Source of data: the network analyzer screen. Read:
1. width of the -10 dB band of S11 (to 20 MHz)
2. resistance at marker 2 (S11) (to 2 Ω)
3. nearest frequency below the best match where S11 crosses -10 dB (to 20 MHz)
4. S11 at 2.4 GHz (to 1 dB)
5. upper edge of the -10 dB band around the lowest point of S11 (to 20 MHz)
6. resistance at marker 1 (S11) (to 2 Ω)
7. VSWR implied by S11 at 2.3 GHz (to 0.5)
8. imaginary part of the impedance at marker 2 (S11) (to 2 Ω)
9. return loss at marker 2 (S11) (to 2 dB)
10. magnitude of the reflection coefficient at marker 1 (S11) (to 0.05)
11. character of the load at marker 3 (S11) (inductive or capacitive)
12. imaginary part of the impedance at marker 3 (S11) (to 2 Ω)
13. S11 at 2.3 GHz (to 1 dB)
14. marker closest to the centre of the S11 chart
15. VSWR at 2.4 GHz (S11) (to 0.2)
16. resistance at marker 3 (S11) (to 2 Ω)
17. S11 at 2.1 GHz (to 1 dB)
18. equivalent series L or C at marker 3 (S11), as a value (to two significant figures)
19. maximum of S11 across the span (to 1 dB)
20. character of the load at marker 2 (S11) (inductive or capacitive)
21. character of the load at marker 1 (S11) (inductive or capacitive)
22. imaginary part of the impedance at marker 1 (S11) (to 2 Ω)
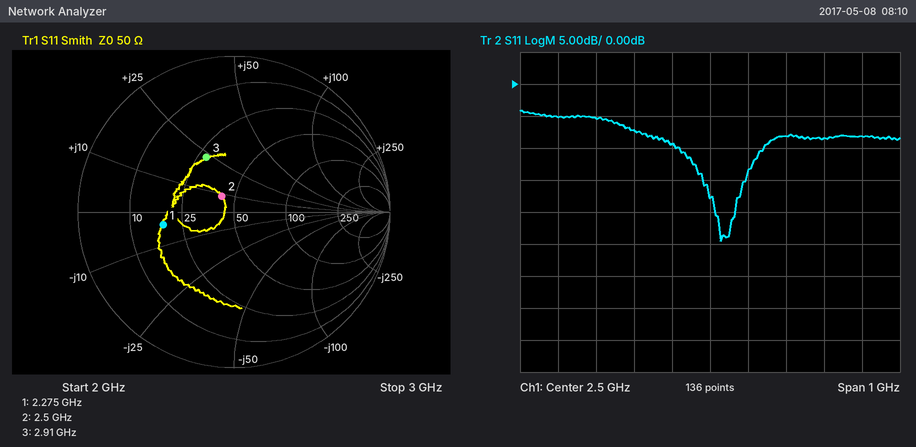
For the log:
220 MHz
42 Ω
2.42 GHz
-9 dB
2.64 GHz
18 Ω
2.5
+8 Ω
18 dB
0.45
inductive
+24 Ω
-7 dB
marker 2
2.0
28 Ω
-5 dB
1.3 nH
-4 dB
inductive
capacitive
-4 Ω
